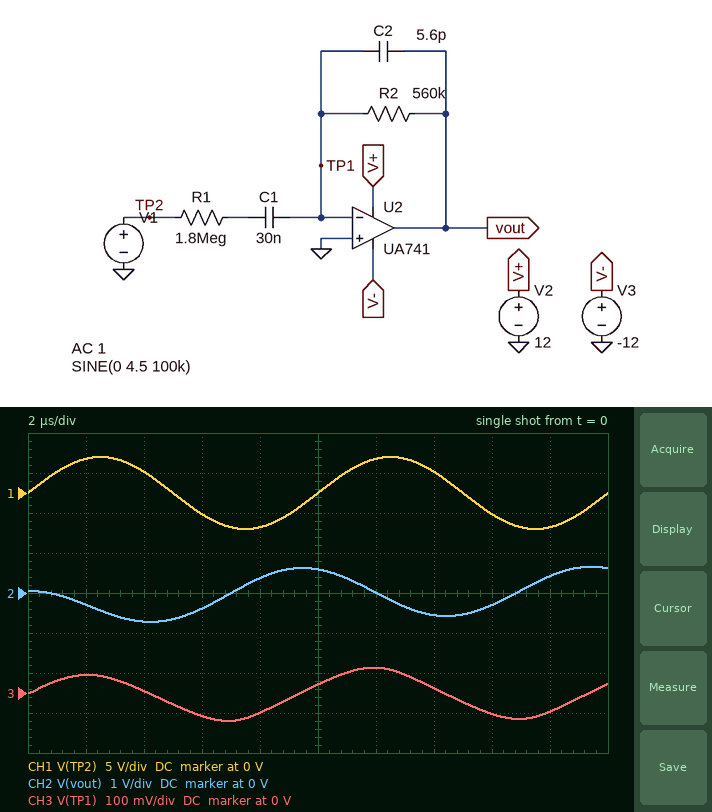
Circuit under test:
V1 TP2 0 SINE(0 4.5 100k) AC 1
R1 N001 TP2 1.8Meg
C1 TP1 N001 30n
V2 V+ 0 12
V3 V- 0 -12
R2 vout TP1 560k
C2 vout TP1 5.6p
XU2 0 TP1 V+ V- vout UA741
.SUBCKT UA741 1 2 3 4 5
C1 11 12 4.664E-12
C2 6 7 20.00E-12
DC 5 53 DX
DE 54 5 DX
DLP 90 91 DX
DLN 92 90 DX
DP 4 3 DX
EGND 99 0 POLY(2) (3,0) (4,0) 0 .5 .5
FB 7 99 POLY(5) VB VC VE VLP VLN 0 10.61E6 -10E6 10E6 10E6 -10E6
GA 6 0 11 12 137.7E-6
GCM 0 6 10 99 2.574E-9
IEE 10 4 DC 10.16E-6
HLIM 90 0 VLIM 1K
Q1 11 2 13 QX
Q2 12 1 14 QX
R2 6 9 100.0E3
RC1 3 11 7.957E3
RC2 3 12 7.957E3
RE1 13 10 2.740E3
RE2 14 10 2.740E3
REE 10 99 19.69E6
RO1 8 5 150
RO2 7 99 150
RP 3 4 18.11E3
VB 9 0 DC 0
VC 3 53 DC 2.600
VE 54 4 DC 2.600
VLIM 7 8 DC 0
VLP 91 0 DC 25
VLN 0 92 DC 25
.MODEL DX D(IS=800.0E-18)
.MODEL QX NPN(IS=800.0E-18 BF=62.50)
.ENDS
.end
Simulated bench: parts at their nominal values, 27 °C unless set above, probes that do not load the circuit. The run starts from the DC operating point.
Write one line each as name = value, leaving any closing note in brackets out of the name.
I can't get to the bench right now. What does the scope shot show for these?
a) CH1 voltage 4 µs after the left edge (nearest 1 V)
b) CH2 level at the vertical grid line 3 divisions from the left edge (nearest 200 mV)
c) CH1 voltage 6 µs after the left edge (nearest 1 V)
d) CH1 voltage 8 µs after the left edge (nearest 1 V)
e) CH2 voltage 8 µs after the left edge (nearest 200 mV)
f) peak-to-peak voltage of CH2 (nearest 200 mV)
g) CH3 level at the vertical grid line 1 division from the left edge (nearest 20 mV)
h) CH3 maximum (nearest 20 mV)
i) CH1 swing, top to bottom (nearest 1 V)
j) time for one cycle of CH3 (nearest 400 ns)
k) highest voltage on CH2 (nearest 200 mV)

CH1 voltage 4 µs after the left edge = 3 V
CH2 level at the vertical grid line 3 divisions from the left edge = -400 mV
CH1 voltage 6 µs after the left edge = -3 V
CH1 voltage 8 µs after the left edge = -4 V
CH2 voltage 8 µs after the left edge = 400 mV
peak-to-peak voltage of CH2 = 1.4 V
CH3 level at the vertical grid line 1 division from the left edge = 40 mV
CH3 maximum = 60 mV
CH1 swing, top to bottom = 9 V
time for one cycle of CH3 = 10.0 µs
highest voltage on CH2 = 600 mV
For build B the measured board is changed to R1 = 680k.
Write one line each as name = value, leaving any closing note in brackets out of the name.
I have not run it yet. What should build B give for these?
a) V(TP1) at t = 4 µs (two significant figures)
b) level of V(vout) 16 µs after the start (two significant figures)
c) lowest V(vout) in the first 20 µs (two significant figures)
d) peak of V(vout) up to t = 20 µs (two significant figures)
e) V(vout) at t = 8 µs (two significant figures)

V(TP1) at t = 4 µs = 84 mV
level of V(vout) 16 µs after the start = -860 mV
lowest V(vout) in the first 20 µs = -1.9 V
peak of V(vout) up to t = 20 µs = 1.3 V
V(vout) at t = 8 µs = -120 mV
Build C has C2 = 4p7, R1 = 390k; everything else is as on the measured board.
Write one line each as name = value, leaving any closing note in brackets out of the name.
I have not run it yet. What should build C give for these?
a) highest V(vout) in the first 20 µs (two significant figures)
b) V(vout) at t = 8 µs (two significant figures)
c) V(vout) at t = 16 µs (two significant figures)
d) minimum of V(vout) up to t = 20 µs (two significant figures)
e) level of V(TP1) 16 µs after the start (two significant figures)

highest V(vout) in the first 20 µs = 750 mV
V(vout) at t = 8 µs = -810 mV
V(vout) at t = 16 µs = -1.4 V
minimum of V(vout) up to t = 20 µs = -2.4 V
level of V(TP1) 16 µs after the start = -650 mV
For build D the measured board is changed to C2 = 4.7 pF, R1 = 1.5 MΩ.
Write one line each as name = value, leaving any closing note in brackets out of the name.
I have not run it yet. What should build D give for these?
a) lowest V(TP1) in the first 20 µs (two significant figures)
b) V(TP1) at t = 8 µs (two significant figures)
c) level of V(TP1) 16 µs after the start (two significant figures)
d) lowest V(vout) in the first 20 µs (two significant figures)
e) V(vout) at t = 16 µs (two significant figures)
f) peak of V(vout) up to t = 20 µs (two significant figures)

lowest V(TP1) in the first 20 µs = -130 mV
V(TP1) at t = 8 µs = -79 mV
level of V(TP1) 16 µs after the start = -82 mV
lowest V(vout) in the first 20 µs = -960 mV
V(vout) at t = 16 µs = -380 mV
peak of V(vout) up to t = 20 µs = 880 mV
